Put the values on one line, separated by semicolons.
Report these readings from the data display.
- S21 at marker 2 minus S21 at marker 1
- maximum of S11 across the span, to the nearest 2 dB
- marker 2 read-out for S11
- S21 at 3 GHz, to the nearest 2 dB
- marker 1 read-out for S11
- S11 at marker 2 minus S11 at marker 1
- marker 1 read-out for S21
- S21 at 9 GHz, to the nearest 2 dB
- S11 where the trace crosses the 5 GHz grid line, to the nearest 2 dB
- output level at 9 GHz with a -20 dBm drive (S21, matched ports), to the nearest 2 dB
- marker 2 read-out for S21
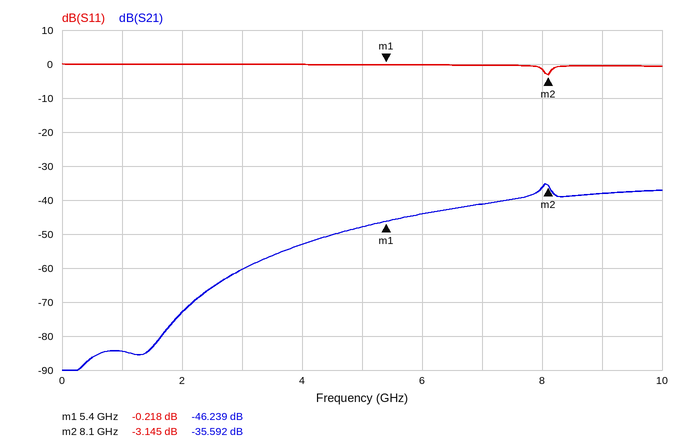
10.647 dB; 0 dB; -3.145 dB; -60 dB; -0.218 dB; -2.927 dB; -46.239 dB; -38 dB; 0 dB; -58 dBm; -35.592 dB
